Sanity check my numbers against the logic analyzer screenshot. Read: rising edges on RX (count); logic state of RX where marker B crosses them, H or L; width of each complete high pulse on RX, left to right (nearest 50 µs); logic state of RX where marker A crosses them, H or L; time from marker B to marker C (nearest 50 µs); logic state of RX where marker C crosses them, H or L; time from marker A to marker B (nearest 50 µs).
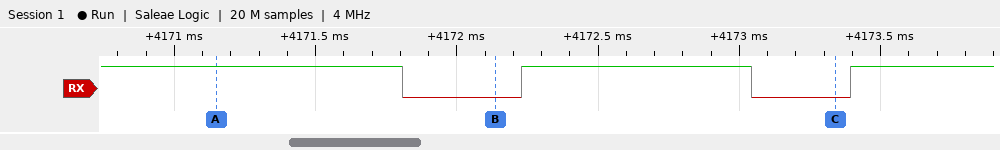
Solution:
2
RX=L
800 µs
RX=H
1200 µs
RX=L
1000 µs
